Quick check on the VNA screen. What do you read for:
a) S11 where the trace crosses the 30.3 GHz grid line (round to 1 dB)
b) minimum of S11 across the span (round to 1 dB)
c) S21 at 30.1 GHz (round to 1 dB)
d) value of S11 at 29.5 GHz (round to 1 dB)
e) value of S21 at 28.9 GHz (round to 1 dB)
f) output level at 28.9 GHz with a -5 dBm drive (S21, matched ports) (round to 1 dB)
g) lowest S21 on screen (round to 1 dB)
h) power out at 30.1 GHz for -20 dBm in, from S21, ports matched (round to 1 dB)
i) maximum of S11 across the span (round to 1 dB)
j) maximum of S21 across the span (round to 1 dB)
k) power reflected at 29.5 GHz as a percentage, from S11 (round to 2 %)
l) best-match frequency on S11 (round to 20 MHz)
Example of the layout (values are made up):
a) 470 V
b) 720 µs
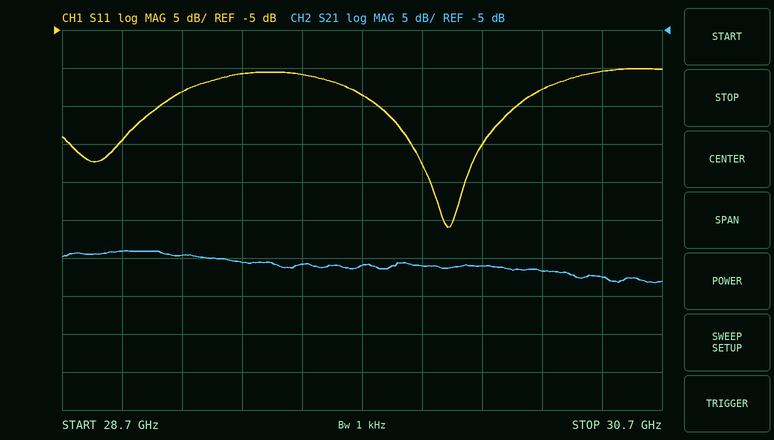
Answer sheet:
a) -13 dB
b) -31 dB
c) -36 dB
d) -11 dB
e) -34 dB
f) -39 dBm
g) -38 dB
h) -56 dBm
i) -10 dB
j) -34 dB
k) 8 %
l) 29.98 GHz
